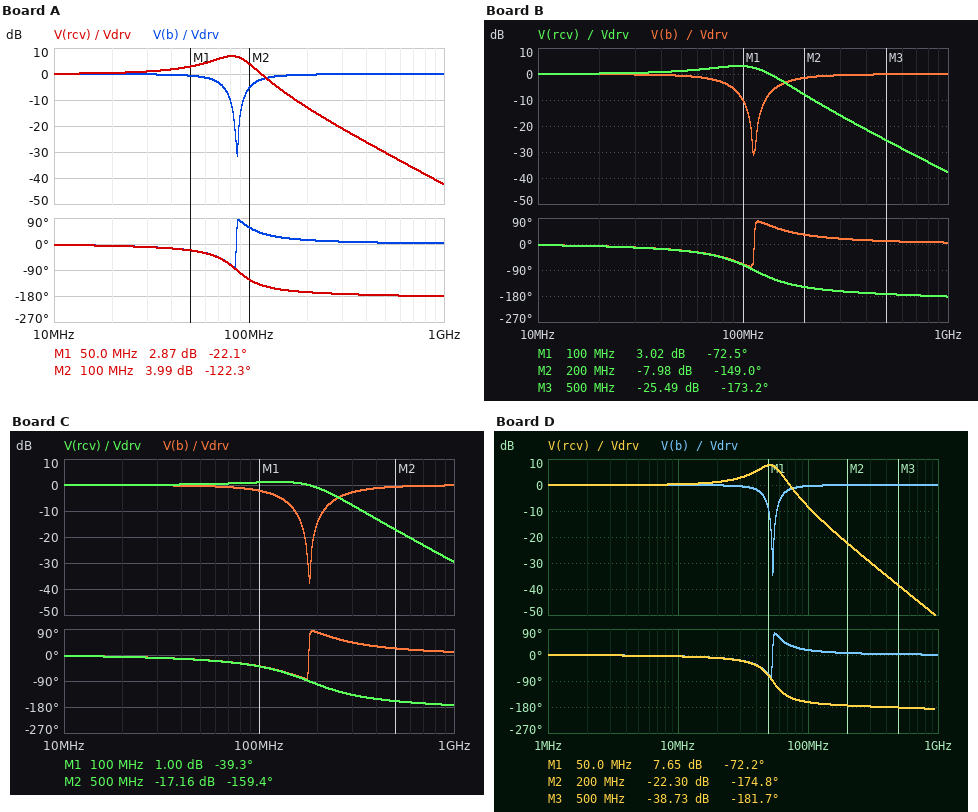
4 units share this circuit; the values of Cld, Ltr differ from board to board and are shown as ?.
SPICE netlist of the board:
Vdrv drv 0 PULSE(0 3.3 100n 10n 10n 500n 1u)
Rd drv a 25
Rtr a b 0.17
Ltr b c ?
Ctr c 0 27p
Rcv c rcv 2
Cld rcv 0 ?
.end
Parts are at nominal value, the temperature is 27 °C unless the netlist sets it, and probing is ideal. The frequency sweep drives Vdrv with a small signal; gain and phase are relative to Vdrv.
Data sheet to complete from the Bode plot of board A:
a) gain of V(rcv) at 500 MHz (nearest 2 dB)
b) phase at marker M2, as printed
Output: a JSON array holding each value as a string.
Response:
["-30 dB", "-122.3 deg"]
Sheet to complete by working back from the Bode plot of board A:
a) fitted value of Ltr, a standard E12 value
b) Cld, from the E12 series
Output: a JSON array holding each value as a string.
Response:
["100 nH", "6.8 pF"]
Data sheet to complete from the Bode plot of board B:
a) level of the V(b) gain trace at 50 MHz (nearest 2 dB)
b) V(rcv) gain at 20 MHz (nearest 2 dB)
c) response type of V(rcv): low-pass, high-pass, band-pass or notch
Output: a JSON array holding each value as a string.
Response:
["0 dB", "0 dB", "low-pass"]
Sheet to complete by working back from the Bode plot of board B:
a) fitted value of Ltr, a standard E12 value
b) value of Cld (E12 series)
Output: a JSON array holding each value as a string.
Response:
["47 nH", "15 pF"]
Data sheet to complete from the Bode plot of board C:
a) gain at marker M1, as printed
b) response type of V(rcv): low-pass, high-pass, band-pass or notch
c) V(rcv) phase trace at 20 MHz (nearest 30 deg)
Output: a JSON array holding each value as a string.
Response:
["1.00 dB", "low-pass", "0 deg"]
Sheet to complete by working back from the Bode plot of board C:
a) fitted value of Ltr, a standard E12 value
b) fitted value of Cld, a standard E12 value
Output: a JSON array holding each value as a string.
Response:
["22 nH", "8.2 pF"]
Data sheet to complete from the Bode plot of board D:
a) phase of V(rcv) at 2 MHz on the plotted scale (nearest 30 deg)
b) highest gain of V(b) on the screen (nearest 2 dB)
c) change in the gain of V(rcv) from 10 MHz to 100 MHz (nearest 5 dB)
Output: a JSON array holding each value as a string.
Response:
["0 deg", "0 dB", "-10 dB"]
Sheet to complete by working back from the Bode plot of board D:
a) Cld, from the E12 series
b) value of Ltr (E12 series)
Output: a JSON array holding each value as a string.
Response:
["22 pF", "180 nH"]
